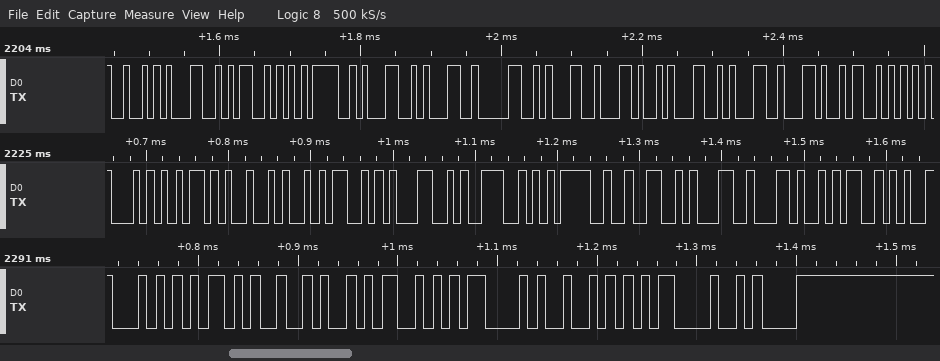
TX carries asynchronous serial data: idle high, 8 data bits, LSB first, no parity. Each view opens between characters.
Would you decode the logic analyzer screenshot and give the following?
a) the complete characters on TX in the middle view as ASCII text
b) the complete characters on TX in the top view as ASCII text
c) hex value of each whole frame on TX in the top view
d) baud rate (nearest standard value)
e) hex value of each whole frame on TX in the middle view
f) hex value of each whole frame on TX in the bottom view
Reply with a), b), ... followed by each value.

a) "T+JSLN=21,M"
b) "RLS=1101,11,S"
c) 52, 4C, 53, 3D, 31, 31, 30, 31, 2C, 31, 31, 2C, 53
d) 115200 baud
e) 54, 2B, 4A, 53, 4C, 4E, 3D, 32, 31, 2C, 4D
f) 54, 2B, 4A, 53, 43, 52, 0D, 0A
